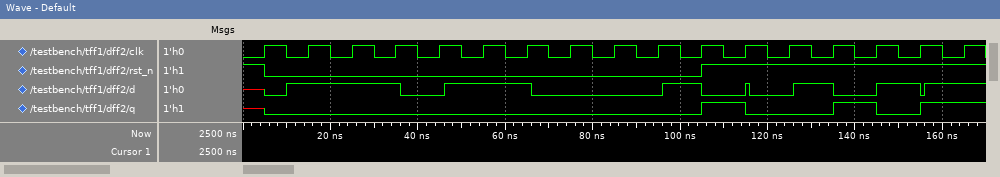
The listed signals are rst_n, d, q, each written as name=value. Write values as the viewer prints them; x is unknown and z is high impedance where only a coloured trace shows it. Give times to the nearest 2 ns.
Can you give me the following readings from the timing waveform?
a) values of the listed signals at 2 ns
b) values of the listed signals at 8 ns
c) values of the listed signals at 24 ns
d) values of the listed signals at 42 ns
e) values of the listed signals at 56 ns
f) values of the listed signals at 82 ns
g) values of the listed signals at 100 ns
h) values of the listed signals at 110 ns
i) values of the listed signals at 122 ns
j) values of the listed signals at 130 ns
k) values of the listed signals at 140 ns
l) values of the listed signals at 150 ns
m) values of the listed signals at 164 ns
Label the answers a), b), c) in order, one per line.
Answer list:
a) rst_n=1, d=x, q=x
b) rst_n=0, d=0, q=0
c) rst_n=0, d=1, q=0
d) rst_n=0, d=0, q=0
e) rst_n=0, d=1, q=0
f) rst_n=0, d=0, q=0
g) rst_n=0, d=1, q=0
h) rst_n=1, d=0, q=1
i) rst_n=1, d=0, q=0
j) rst_n=1, d=1, q=0
k) rst_n=1, d=0, q=1
l) rst_n=1, d=1, q=0
m) rst_n=1, d=1, q=1
